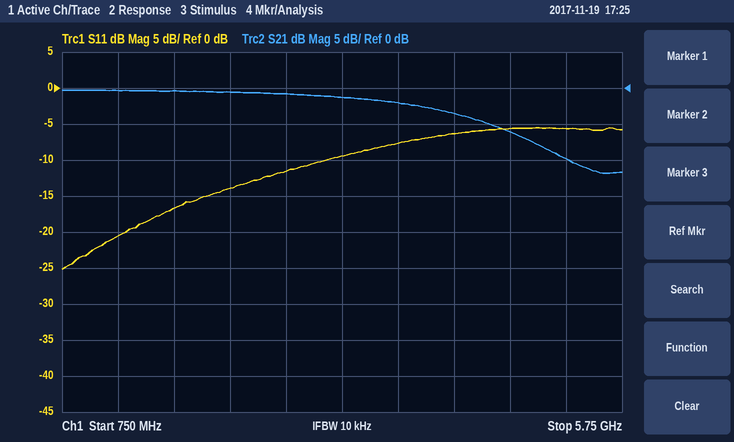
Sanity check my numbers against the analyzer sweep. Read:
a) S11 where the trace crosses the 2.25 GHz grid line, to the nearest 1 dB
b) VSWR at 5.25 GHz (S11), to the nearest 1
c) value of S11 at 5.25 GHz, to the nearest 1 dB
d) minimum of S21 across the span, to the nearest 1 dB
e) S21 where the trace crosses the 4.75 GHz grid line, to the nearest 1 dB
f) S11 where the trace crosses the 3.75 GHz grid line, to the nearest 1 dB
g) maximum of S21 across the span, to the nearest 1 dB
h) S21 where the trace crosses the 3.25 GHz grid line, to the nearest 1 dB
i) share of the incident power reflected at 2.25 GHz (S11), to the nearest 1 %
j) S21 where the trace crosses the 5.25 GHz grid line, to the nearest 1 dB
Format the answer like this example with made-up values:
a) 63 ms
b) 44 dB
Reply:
a) -14 dB
b) 3
c) -6 dB
d) -12 dB
e) -6 dB
f) -8 dB
g) 0 dB
h) -1 dB
i) 4 %
j) -10 dB
